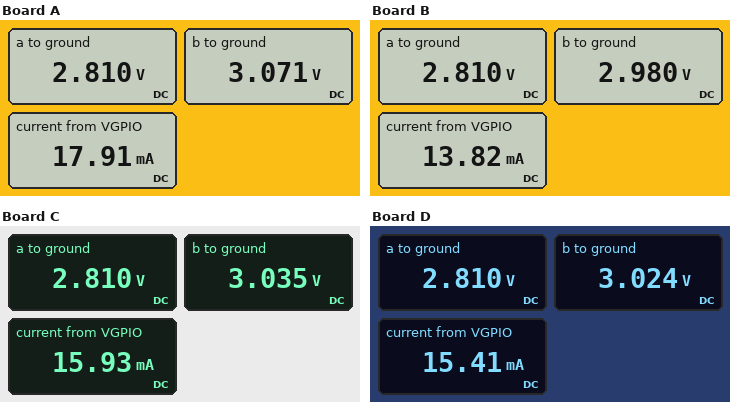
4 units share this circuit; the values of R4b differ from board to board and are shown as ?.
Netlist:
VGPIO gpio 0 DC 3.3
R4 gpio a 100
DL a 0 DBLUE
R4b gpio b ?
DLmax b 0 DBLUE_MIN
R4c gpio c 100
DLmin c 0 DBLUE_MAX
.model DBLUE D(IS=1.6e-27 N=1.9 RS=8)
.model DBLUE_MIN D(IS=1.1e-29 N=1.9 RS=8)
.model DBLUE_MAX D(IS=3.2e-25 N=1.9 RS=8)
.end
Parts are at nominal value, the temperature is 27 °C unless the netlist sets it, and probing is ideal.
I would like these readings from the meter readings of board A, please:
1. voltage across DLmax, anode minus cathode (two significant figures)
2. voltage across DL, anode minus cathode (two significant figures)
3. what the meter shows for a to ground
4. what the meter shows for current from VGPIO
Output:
3.1 V
2.8 V
2.810 V
17.91 mA
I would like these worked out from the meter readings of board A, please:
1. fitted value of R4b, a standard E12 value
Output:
39 Ω
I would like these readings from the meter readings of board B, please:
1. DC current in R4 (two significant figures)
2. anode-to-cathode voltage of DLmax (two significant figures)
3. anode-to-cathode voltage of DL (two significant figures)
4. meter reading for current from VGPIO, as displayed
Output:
4.9 mA
3.0 V
2.8 V
13.82 mA
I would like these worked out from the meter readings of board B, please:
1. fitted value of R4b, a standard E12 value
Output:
180 Ω
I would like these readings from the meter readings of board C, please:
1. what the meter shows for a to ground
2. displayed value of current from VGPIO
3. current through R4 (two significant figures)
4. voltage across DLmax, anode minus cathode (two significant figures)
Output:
2.810 V
15.93 mA
4.9 mA
3.0 V
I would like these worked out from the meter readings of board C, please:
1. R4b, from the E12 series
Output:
68 Ω
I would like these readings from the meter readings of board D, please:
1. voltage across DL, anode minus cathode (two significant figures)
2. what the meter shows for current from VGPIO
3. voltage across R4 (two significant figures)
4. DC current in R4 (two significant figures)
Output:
2.8 V
15.41 mA
490 mV
4.9 mA
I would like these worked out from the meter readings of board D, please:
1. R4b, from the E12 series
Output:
82 Ω
